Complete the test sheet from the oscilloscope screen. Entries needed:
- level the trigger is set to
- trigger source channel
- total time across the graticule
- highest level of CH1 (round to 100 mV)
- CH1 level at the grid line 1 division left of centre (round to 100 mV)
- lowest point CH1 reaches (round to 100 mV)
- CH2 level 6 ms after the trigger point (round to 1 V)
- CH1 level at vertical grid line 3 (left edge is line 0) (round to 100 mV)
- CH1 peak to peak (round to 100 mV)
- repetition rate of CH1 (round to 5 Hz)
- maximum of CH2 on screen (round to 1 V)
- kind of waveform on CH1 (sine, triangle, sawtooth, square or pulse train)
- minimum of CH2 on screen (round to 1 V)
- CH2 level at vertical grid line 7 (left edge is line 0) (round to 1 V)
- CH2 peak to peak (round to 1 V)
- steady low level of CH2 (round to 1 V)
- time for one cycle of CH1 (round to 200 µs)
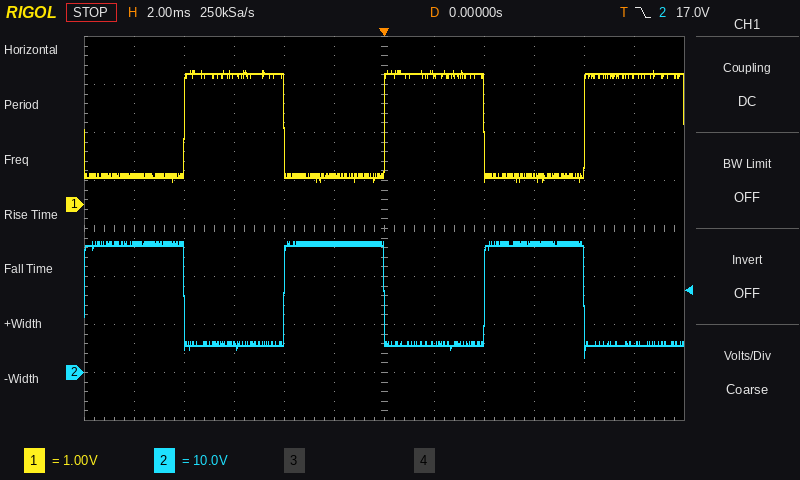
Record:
17.0 V
CH2
24 ms
2.8 V
600 mV
500 mV
27 V
2.7 V
2.3 V
125 Hz
27 V
square
3 V
6 V
24 V
6 V
8.0 ms
